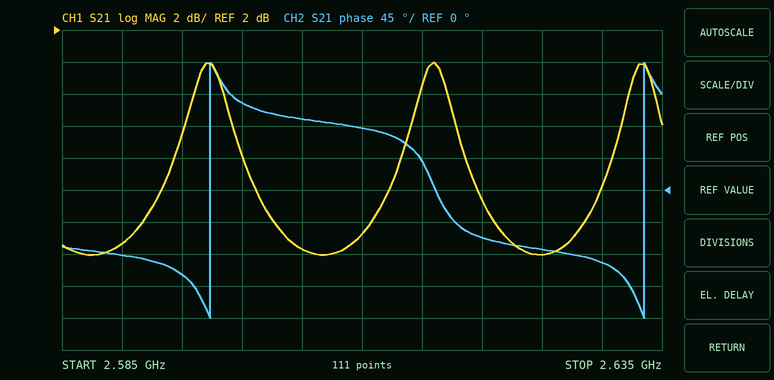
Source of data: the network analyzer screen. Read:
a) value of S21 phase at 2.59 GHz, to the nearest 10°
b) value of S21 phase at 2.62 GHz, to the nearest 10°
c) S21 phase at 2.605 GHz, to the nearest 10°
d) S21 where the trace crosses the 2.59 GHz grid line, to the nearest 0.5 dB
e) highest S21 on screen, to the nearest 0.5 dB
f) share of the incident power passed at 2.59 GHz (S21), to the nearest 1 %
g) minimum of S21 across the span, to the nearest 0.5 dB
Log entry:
-90°
-70°
100°
-11.5 dB
0.0 dB
7 %
-12.0 dB
